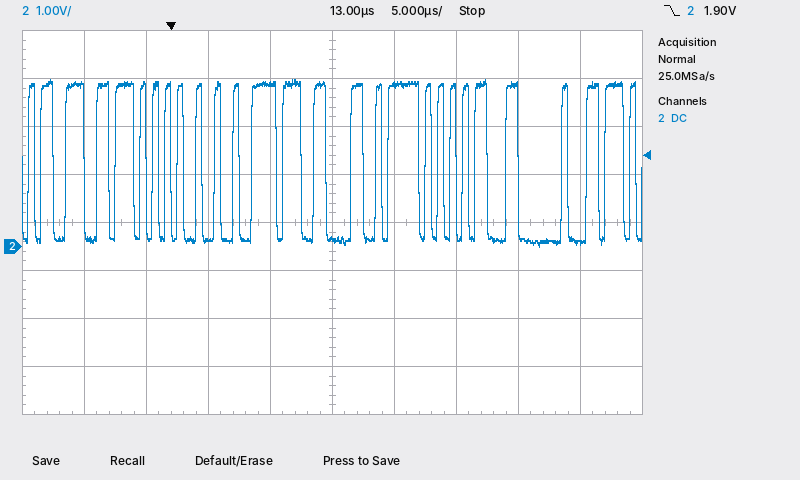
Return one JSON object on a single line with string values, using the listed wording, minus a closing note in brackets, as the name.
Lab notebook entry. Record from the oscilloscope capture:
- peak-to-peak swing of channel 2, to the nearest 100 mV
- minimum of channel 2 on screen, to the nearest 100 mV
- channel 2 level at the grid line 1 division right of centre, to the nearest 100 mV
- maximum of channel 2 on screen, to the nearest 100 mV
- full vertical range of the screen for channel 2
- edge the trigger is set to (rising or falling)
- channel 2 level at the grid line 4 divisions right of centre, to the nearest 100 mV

{"peak-to-peak swing of channel 2, to the nearest 100 mV": "3.5 V", "minimum of channel 2 on screen, to the nearest 100 mV": "0.0 V", "channel 2 level at the grid line 1 division right of centre, to the nearest 100 mV": "3.4 V", "maximum of channel 2 on screen, to the nearest 100 mV": "3.5 V", "full vertical range of the screen for channel 2": "8 V", "edge the trigger is set to": "falling", "channel 2 level at the grid line 4 divisions right of centre, to the nearest 100 mV": "100 mV"}
